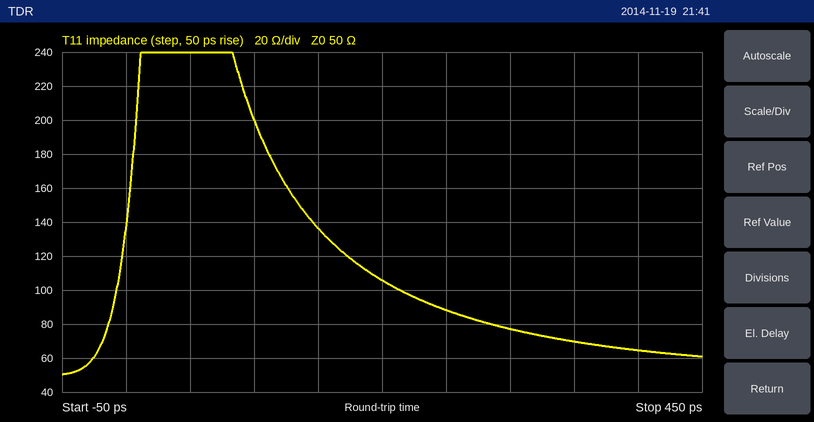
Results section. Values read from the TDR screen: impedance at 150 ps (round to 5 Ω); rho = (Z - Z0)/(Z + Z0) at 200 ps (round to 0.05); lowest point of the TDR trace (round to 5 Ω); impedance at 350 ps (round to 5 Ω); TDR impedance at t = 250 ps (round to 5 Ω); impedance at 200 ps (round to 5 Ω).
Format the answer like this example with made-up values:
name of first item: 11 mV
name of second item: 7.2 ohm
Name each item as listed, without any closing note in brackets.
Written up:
impedance at 150 ps: 135 Ω
rho = (Z - Z0)/(Z + Z0) at 200 ps: +0.35
lowest point of the TDR trace: 50 Ω
impedance at 350 ps: 70 Ω
TDR impedance at t = 250 ps: 90 Ω
impedance at 200 ps: 105 Ω
